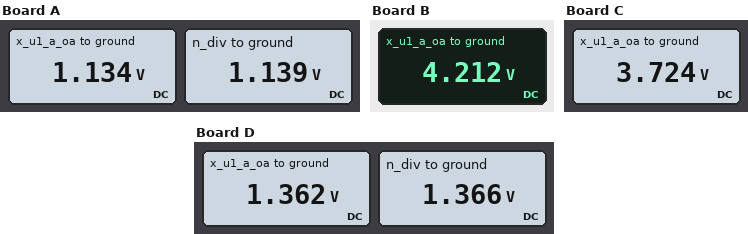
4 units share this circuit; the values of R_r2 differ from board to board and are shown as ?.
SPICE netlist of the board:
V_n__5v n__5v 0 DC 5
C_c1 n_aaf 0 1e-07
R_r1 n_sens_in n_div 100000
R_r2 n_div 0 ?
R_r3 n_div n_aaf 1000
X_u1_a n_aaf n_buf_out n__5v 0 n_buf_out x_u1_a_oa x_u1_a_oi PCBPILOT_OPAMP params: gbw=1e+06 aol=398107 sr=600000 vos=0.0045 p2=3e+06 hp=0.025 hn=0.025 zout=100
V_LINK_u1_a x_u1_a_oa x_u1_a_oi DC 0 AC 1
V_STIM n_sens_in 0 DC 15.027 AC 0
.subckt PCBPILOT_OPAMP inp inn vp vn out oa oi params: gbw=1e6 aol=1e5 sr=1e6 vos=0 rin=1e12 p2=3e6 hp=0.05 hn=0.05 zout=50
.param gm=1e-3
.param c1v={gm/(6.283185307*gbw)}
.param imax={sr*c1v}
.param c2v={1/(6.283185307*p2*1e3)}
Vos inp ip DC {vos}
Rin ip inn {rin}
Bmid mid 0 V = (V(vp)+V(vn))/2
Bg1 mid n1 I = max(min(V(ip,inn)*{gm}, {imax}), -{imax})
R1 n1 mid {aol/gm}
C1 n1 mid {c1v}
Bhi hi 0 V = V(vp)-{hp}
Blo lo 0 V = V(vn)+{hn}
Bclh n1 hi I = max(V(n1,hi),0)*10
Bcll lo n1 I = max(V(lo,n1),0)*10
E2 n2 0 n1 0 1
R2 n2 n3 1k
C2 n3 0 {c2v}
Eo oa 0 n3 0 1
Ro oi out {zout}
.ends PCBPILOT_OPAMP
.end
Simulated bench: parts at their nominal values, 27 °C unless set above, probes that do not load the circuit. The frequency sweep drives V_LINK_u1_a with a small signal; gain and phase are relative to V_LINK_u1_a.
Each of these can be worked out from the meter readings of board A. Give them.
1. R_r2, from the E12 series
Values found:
8.2 kΩ
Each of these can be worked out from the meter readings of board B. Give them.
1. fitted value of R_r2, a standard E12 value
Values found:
39 kΩ
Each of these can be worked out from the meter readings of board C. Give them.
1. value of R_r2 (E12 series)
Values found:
33 kΩ
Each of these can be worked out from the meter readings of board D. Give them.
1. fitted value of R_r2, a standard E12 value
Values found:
10 kΩ
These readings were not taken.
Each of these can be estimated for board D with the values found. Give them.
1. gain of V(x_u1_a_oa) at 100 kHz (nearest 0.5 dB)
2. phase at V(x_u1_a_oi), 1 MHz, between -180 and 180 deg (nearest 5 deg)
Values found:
0 dB
-130 deg
